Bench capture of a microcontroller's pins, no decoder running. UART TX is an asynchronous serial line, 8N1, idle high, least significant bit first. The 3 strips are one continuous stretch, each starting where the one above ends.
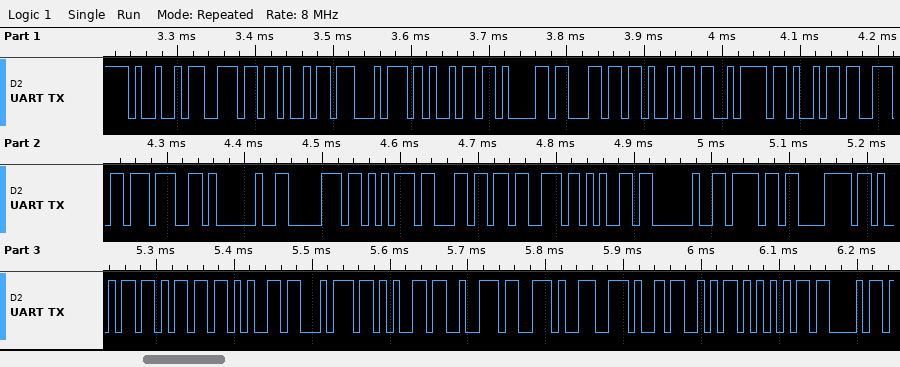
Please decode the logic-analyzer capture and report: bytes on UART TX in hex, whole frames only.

0x49 0x6E 0x69 0x74 0x69 0x61 0x6C 0x69 0x7A 0x69 0x6E 0x67 0x20 0x70 0x75 0x6C 0x73 0x65 0x20 0x6F 0x78 0x69 0x6D 0x65 0x74 0x65 0x72 0x2E 0x2E 0x53 0x55 0x43
